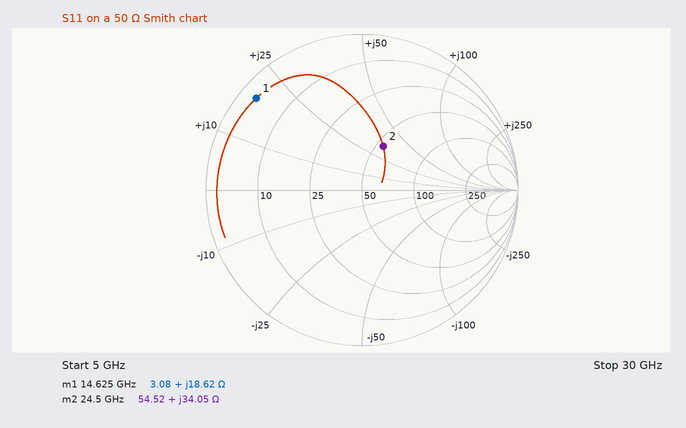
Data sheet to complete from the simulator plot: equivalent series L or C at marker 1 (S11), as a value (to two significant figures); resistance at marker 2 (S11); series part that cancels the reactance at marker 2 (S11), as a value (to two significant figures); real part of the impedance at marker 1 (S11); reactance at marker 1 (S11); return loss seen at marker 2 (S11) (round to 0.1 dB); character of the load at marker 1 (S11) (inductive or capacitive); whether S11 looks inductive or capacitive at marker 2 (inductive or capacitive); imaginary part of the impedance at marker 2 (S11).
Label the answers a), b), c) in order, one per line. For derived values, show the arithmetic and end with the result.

a) L = 18.62 Ω/(2π × 14.625 GHz) ≈ 203 pH, so 200 pH to two significant figures
b) 54.52 Ω
c) C = 1/(2π × 24.5 GHz × 34.05 Ω) ≈ 191 fF, so 190 fF to two significant figures
d) 3.08 Ω
e) +18.62 Ω
f) 10.1 dB
g) inductive
h) inductive
i) +34.05 Ω
